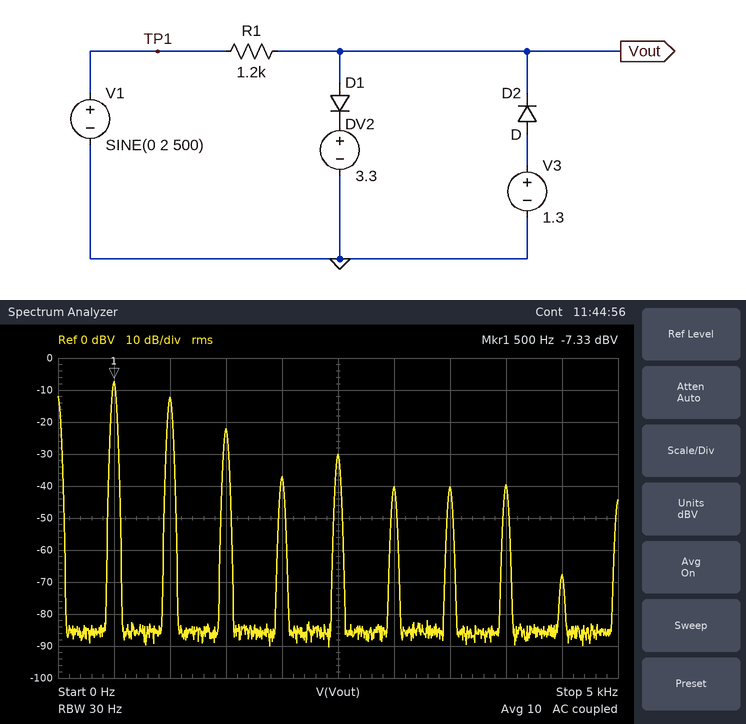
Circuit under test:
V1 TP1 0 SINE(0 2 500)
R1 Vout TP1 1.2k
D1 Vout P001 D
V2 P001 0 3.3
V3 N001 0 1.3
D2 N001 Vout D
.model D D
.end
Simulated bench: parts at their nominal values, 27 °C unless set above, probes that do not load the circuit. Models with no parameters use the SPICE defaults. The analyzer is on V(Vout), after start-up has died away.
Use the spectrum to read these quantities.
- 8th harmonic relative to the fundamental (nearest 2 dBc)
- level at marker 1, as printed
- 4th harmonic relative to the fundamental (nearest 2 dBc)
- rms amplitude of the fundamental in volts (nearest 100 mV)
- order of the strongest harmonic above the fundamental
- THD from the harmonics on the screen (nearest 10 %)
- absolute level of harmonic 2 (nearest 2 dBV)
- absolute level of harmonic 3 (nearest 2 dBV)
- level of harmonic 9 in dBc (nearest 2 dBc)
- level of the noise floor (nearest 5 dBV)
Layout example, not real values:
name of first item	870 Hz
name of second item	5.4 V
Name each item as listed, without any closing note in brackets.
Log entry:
8th harmonic relative to the fundamental	-32 dBc
level at marker 1, as printed	-7.33 dBV
4th harmonic relative to the fundamental	-30 dBc
rms amplitude of the fundamental in volts	400 mV
order of the strongest harmonic above the fundamental	2
THD from the harmonics on the screen	60 %
absolute level of harmonic 2	-12 dBV
absolute level of harmonic 3	-22 dBV
level of harmonic 9 in dBc	-60 dBc
level of the noise floor	-85 dBV
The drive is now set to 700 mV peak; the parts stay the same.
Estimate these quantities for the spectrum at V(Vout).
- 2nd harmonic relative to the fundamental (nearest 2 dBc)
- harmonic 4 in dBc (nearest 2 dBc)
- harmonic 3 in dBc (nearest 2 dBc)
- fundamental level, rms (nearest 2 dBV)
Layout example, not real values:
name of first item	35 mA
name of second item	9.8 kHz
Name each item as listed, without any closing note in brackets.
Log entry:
2nd harmonic relative to the fundamental	-10 dBc
harmonic 4 in dBc	-22 dBc
harmonic 3 in dBc	-16 dBc
fundamental level, rms	-32 dBV
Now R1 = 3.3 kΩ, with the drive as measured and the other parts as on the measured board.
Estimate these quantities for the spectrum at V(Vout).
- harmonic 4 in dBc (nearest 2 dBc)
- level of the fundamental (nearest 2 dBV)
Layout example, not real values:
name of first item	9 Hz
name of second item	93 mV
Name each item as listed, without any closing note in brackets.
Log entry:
harmonic 4 in dBc	-32 dBc
level of the fundamental	-8 dBV
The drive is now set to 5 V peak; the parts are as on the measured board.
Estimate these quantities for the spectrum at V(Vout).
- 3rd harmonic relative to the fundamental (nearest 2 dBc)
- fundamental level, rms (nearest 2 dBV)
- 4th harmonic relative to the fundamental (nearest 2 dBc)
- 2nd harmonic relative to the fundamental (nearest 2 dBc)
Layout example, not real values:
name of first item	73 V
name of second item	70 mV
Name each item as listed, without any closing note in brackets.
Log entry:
3rd harmonic relative to the fundamental	-30 dBc
fundamental level, rms	2 dBV
4th harmonic relative to the fundamental	-16 dBc
2nd harmonic relative to the fundamental	-8 dBc
